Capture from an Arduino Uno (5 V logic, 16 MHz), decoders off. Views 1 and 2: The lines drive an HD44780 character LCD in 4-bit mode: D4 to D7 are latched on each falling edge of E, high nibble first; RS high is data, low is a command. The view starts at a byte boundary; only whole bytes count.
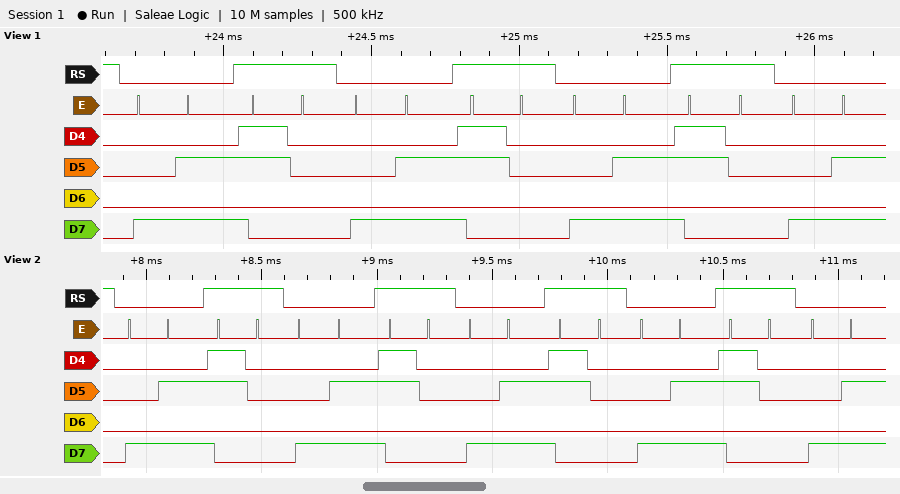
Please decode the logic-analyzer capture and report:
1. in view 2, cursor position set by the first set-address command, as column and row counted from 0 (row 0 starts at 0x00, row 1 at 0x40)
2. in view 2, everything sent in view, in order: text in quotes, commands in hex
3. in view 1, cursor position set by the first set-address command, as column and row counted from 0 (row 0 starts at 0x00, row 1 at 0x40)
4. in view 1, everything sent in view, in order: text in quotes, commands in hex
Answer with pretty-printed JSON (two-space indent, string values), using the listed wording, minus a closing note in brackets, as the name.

{
  "in view 2, cursor position set by the first set-address command, as column and row counted from 0": "column 10, row 0",
  "in view 2, everything sent in view, in order: text in quotes, commands in hex": "0x8A \"0\" 0x8A \"0\" 0x8A \"0\" 0x8A \"0\" 0x8A",
  "in view 1, cursor position set by the first set-address command, as column and row counted from 0": "column 10, row 0",
  "in view 1, everything sent in view, in order: text in quotes, commands in hex": "0x8A \"0\" 0x8A \"0\" 0x8A \"0\" 0x8A"
}
